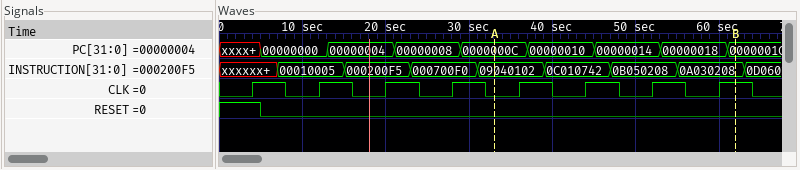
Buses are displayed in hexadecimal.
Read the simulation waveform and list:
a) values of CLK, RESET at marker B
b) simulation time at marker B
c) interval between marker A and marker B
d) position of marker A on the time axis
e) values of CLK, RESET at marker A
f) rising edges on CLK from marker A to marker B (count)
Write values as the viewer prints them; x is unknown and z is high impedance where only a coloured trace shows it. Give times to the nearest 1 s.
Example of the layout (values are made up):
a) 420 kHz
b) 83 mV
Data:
a) CLK=1, RESET=0
b) 62 s
c) 29 s
d) 33 s
e) CLK=0, RESET=0
f) 4
